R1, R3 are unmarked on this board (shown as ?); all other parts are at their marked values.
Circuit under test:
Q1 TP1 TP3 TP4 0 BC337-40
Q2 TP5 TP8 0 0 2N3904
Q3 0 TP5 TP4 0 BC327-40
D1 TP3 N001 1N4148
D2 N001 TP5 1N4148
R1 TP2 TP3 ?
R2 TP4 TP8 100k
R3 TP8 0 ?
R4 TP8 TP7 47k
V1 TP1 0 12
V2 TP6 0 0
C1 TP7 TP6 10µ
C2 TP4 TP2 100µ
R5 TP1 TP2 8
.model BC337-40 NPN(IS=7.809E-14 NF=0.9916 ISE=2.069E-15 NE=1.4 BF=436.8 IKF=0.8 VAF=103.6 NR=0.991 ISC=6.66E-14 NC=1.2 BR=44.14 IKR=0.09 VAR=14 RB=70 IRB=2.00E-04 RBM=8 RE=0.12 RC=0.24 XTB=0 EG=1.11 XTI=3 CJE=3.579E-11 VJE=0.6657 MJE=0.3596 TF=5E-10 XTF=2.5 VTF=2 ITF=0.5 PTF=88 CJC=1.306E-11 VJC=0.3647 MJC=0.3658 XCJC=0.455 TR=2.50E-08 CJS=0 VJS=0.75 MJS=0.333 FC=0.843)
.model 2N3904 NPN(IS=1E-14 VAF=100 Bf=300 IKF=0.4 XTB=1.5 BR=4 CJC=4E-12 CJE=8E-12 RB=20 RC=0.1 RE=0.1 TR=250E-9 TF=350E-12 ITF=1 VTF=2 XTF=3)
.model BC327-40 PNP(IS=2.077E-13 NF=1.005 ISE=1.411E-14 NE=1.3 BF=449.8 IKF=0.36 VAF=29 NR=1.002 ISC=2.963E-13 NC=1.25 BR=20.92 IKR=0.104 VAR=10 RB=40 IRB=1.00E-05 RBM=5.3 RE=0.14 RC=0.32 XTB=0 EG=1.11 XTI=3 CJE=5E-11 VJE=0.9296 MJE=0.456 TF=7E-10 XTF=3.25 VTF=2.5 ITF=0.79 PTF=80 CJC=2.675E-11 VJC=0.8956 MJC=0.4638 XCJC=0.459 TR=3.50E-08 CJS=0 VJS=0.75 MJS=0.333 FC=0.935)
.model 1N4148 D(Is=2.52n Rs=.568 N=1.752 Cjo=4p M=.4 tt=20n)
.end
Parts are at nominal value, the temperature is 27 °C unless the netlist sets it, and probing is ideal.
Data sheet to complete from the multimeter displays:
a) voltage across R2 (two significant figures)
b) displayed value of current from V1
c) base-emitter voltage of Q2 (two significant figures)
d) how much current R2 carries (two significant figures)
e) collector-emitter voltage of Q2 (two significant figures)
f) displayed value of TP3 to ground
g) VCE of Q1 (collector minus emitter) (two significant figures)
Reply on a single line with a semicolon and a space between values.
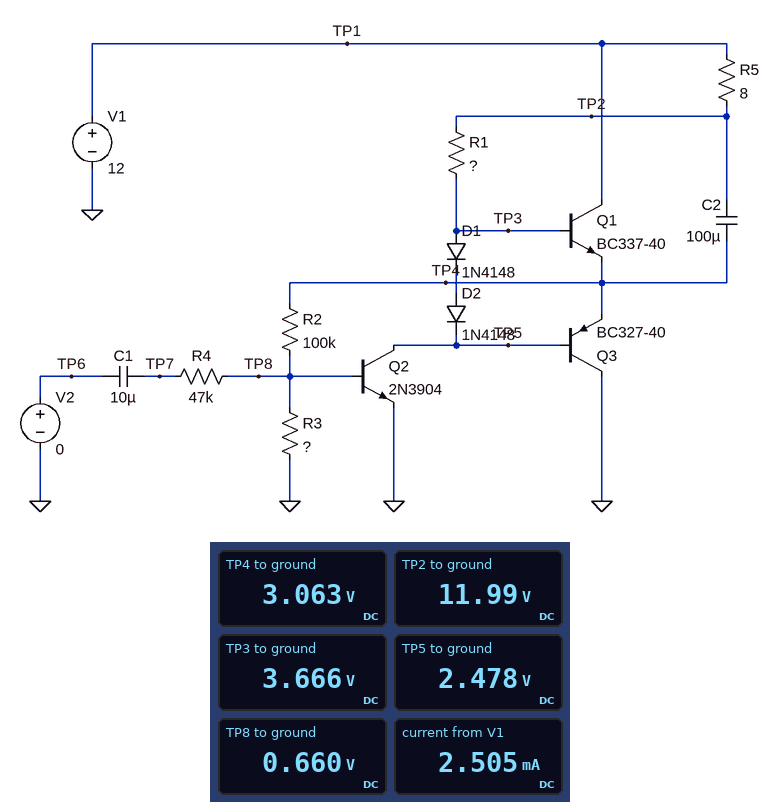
2.4 V; 2.505 mA; 660 mV; 24 µA; 2.5 V; 3.666 V; 8.9 V
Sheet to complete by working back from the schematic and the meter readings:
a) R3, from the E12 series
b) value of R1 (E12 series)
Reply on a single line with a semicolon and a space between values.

33 kΩ; 6.8 kΩ
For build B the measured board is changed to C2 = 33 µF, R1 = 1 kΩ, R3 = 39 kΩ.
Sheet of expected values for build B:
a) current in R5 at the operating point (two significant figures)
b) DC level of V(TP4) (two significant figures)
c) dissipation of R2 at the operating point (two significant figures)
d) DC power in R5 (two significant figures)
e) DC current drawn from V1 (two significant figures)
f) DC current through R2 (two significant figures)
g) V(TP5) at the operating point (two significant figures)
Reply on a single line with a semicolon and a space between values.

6.6 mA; 4.7 V; 160 µW; 350 µW; 29 mA; 40 µA; 4.0 V
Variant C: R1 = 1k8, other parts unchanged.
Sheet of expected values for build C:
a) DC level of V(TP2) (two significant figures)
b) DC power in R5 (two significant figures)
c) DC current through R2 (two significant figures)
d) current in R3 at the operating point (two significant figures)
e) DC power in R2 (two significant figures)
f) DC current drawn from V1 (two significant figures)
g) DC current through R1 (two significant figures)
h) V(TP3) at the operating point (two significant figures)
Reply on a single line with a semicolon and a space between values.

12 V; 130 µW; 34 µA; 21 µA; 120 µW; 14 mA; 4.0 mA; 4.8 V
